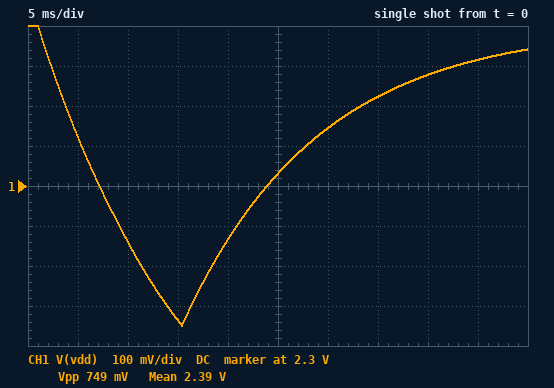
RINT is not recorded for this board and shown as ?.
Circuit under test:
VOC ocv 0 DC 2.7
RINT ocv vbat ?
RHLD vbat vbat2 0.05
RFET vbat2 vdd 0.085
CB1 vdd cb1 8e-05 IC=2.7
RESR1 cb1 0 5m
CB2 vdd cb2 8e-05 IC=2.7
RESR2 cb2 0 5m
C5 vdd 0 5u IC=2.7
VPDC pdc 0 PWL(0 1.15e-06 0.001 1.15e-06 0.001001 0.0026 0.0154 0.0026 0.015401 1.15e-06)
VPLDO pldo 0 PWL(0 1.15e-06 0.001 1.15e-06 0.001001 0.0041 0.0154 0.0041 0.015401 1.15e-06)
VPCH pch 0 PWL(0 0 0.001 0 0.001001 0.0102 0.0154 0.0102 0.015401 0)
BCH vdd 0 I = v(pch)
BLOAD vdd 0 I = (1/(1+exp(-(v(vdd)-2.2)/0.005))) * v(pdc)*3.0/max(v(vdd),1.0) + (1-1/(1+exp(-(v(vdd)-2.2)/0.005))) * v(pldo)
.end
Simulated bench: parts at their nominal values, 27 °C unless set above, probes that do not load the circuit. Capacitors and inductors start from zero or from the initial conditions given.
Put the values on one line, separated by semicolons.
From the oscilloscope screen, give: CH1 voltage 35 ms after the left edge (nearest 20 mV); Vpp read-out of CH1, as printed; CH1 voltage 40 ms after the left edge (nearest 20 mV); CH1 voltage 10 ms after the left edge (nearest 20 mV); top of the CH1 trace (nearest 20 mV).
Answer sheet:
2.52 V; 749 mV; 2.58 V; 2.16 V; 2.70 V
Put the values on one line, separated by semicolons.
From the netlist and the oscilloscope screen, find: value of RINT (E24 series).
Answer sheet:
82 Ω
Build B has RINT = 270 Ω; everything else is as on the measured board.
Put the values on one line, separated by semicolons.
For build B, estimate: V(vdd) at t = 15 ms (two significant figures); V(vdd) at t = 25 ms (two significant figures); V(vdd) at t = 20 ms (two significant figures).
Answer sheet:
1.7 V; 1.9 V; 1.8 V
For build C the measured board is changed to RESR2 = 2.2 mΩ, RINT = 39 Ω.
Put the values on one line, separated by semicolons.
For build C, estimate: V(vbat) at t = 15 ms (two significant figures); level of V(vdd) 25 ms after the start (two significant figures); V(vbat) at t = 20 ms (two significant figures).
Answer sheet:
2.2 V; 2.6 V; 2.5 V
